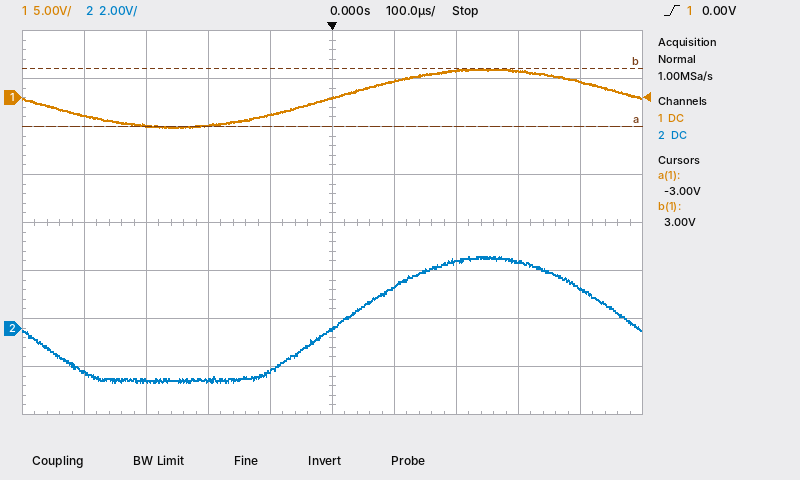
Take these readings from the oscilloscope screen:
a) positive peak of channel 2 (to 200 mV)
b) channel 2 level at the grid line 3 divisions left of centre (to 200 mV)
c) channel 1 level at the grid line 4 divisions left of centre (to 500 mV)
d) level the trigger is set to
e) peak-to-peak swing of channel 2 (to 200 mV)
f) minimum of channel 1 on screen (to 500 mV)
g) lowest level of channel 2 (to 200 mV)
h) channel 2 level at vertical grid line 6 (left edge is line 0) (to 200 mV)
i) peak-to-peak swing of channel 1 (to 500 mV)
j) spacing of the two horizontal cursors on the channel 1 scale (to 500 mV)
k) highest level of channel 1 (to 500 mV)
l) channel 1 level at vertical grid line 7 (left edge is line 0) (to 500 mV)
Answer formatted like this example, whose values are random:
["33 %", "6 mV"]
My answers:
["3.0 V", "-2.2 V", "-2.0 V", "0.00 V", "5.2 V", "-3.0 V", "-2.2 V", "1.8 V", "6.0 V", "6.0 V", "3.0 V", "3.0 V"]
